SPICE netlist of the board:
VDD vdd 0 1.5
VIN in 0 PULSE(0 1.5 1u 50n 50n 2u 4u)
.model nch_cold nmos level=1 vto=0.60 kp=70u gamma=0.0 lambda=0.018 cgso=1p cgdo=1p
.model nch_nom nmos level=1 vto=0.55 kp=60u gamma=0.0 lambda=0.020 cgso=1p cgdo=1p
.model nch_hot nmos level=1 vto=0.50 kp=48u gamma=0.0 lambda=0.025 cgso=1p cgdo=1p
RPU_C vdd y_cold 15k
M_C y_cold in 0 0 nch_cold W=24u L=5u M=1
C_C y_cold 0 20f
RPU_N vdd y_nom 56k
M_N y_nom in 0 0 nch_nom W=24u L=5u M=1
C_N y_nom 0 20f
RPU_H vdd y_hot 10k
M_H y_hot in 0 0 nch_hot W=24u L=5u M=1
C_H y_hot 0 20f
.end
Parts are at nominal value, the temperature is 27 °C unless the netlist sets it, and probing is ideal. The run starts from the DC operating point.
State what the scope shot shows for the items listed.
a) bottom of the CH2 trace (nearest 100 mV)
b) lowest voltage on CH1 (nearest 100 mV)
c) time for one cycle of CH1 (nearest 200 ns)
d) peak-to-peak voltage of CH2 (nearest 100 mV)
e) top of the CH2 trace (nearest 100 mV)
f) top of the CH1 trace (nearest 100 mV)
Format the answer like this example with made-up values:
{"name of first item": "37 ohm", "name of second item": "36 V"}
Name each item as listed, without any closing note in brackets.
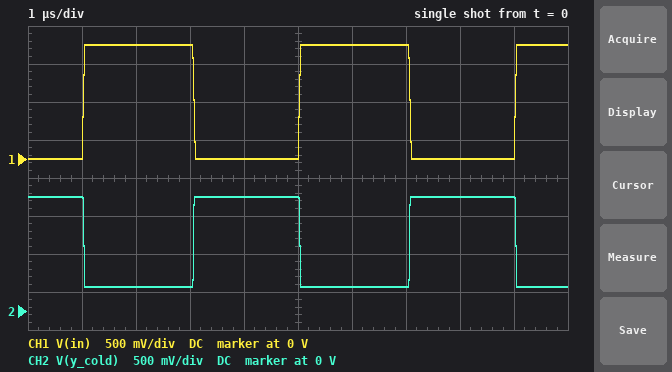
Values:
{"bottom of the CH2 trace": "300 mV", "lowest voltage on CH1": "0 V", "time for one cycle of CH1": "4.0 µs", "peak-to-peak voltage of CH2": "1.2 V", "top of the CH2 trace": "1.5 V", "top of the CH1 trace": "1.5 V"}
